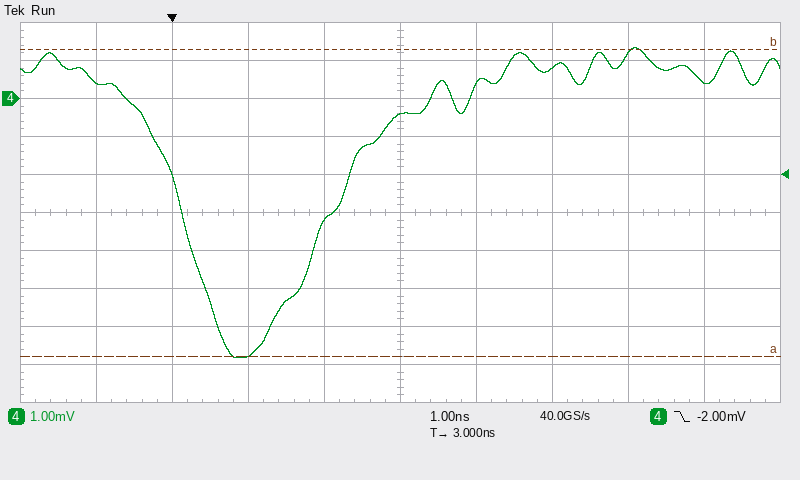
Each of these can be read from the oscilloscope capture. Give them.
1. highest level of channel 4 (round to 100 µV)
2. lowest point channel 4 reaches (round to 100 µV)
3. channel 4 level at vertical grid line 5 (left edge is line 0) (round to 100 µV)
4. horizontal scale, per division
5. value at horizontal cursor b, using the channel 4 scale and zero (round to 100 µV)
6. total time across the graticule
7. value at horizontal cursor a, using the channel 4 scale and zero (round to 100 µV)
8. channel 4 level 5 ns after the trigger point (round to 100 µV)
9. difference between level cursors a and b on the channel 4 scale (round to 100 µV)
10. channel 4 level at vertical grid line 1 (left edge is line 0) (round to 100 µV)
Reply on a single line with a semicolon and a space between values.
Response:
1.3 mV; -6.8 mV; -400 µV; 1 ns; 1.3 mV; 10 ns; -6.8 mV; 800 µV; 8.1 mV; 400 µV
